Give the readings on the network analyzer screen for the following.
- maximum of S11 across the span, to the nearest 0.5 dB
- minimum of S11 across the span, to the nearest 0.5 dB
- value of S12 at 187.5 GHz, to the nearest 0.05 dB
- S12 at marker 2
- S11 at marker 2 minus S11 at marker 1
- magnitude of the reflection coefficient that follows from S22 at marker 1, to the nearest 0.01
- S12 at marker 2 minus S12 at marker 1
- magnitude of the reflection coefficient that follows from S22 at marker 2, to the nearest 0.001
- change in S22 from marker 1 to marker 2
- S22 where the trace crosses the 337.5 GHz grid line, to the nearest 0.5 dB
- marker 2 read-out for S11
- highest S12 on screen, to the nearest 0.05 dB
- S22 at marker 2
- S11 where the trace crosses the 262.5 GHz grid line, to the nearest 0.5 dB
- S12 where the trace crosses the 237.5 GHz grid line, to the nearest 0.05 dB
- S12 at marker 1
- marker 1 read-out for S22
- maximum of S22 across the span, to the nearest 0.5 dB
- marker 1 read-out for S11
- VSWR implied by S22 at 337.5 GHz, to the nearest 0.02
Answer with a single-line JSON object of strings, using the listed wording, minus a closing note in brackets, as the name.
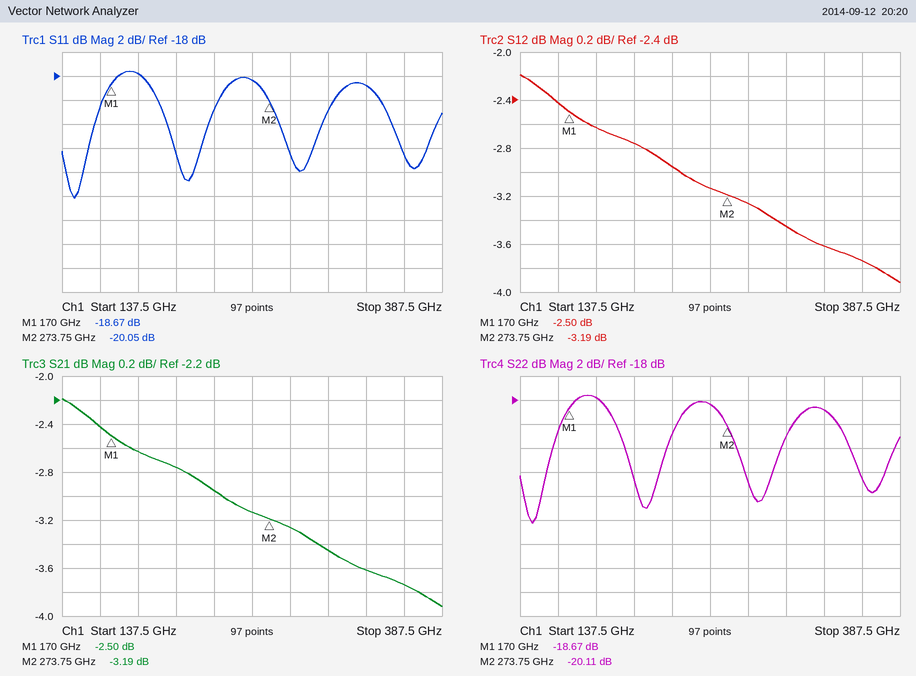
{"maximum of S11 across the span, to the nearest 0.5 dB": "-17.5 dB", "minimum of S11 across the span, to the nearest 0.5 dB": "-28.0 dB", "value of S12 at 187.5 GHz, to the nearest 0.05 dB": "-2.65 dB", "S12 at marker 2": "-3.19 dB", "S11 at marker 2 minus S11 at marker 1": "-1.38 dB", "magnitude of the reflection coefficient that follows from S22 at marker 1, to the nearest 0.01": "0.12", "S12 at marker 2 minus S12 at marker 1": "-0.69 dB", "magnitude of the reflection coefficient that follows from S22 at marker 2, to the nearest 0.001": "0.099", "change in S22 from marker 1 to marker 2": "-1.44 dB", "S22 where the trace crosses the 337.5 GHz grid line, to the nearest 0.5 dB": "-19.0 dB", "marker 2 read-out for S11": "-20.05 dB", "highest S12 on screen, to the nearest 0.05 dB": "-2.20 dB", "S22 at marker 2": "-20.11 dB", "S11 where the trace crosses the 262.5 GHz grid line, to the nearest 0.5 dB": "-18.5 dB", "S12 where the trace crosses the 237.5 GHz grid line, to the nearest 0.05 dB": "-2.95 dB", "S12 at marker 1": "-2.50 dB", "marker 1 read-out for S22": "-18.67 dB", "maximum of S22 across the span, to the nearest 0.5 dB": "-17.5 dB", "marker 1 read-out for S11": "-18.67 dB", "VSWR implied by S22 at 337.5 GHz, to the nearest 0.02": "1.26"}
